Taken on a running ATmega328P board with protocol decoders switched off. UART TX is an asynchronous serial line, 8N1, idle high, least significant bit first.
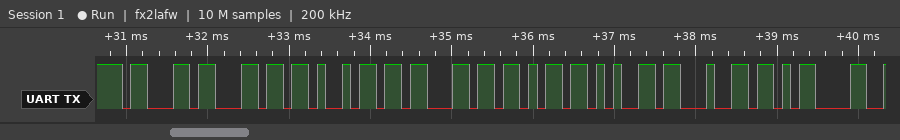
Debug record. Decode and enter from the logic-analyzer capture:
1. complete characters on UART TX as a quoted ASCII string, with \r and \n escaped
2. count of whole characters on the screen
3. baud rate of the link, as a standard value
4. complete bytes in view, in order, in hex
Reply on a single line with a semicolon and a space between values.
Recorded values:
"clicked\r"; 8; 9600 baud; 0x63 0x6C 0x69 0x63 0x6B 0x65 0x64 0x0D
